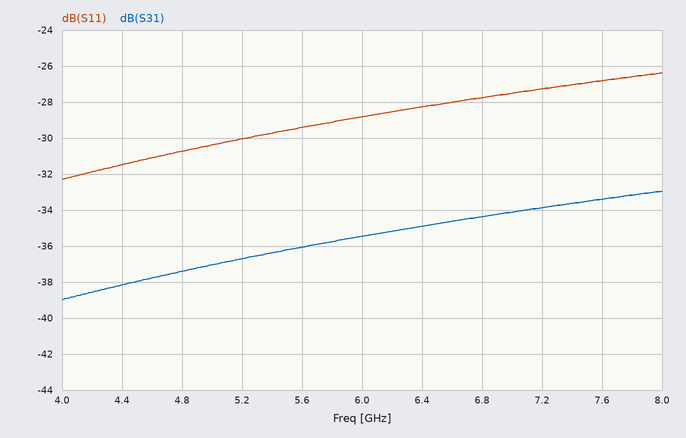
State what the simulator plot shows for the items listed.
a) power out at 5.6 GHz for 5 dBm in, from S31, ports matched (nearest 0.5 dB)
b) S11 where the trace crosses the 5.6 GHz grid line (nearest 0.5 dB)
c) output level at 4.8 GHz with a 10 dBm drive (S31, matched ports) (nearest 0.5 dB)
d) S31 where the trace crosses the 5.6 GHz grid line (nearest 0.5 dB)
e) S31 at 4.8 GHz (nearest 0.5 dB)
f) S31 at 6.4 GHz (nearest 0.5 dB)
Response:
-31.0 dBm
-29.5 dB
-27.5 dBm
-36.0 dB
-37.5 dB
-35.0 dB
